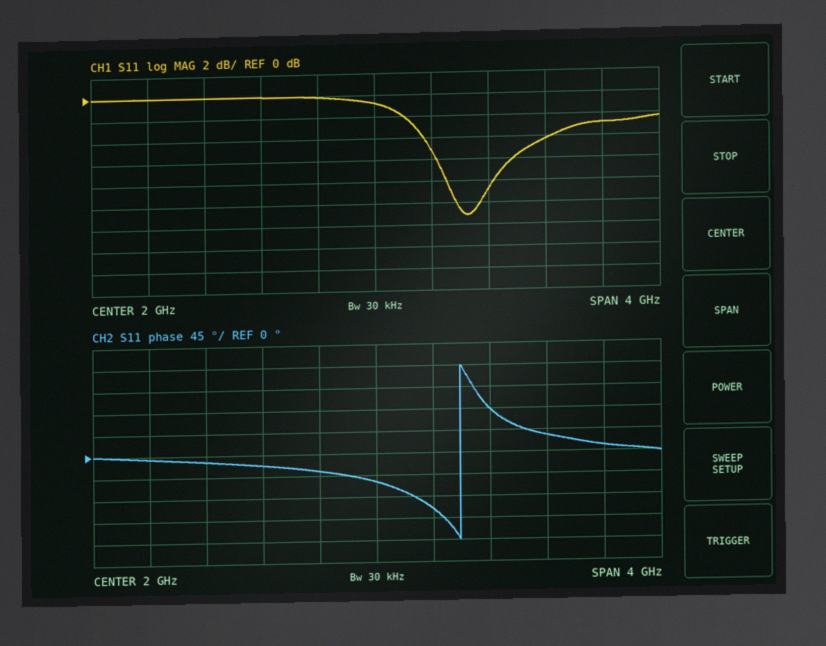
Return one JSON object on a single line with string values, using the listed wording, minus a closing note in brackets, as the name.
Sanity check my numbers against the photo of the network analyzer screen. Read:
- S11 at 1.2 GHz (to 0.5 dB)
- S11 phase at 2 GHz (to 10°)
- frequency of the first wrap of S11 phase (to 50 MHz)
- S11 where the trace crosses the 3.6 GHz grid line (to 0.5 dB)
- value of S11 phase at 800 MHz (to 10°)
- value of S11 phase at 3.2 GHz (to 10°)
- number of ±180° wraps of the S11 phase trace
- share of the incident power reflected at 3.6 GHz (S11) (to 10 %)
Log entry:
{"S11 at 1.2 GHz": "0.0 dB", "S11 phase at 2 GHz": "-60°", "frequency of the first wrap of S11 phase": "2.60 GHz", "S11 where the trace crosses the 3.6 GHz grid line": "-3.0 dB", "value of S11 phase at 800 MHz": "-10°", "value of S11 phase at 3.2 GHz": "30°", "number of ±180° wraps of the S11 phase trace": "1", "share of the incident power reflected at 3.6 GHz (S11)": "50 %"}
